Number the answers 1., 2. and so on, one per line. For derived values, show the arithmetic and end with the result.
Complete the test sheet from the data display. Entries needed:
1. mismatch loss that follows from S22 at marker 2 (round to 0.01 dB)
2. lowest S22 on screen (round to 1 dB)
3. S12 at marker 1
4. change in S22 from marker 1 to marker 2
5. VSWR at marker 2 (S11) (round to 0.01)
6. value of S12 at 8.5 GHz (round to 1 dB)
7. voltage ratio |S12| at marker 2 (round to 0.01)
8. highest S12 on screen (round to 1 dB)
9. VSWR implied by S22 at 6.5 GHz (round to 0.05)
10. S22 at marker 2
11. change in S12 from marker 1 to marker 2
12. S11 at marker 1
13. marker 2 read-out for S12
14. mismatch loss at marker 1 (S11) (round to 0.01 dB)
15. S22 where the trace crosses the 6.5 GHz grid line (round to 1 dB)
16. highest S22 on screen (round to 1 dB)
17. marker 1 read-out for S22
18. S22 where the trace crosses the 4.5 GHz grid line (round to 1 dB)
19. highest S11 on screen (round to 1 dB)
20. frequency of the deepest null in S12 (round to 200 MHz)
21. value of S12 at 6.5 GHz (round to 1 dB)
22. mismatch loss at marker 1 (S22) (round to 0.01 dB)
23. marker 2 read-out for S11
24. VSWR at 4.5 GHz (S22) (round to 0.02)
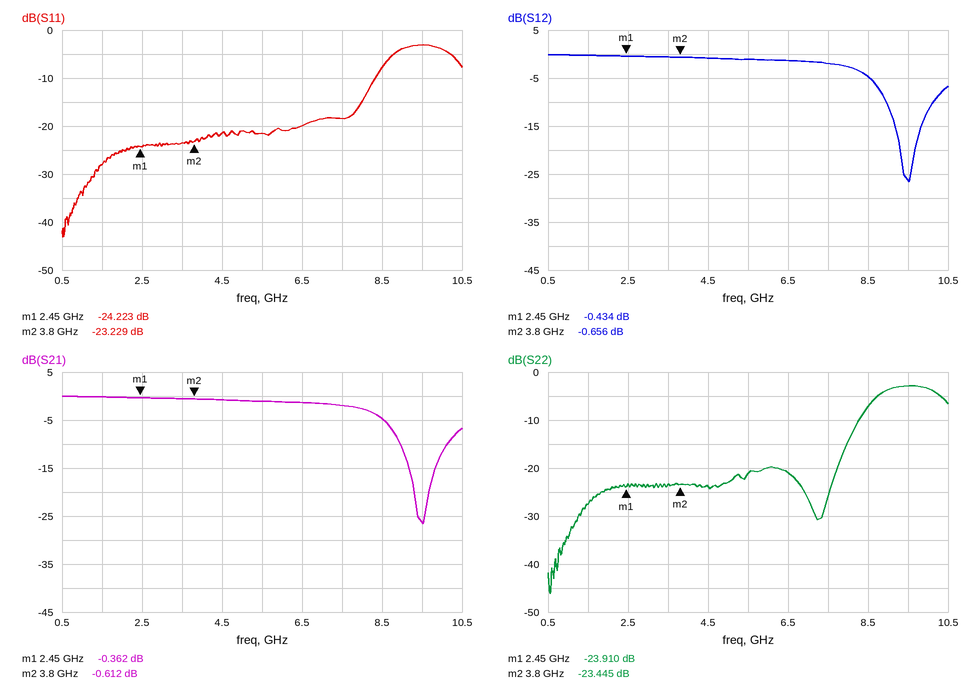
1. −10 log10(1 − 10^(-23.445/10)) ≈ 0.02 dB
2. -46 dB
3. -0.434 dB
4. -23.445 − (-23.91) = 0.465 dB
5. (1 + 0.0690)/(1 − 0.0690) ≈ 1.15
6. -5 dB
7. 10^(-0.656/20) ≈ 0.93
8. 0 dB
9. |Γ| = 10^(-21/20) = 0.0891; VSWR = (1 + 0.0891)/(1 − 0.0891) ≈ 1.20
10. -23.445 dB
11. -0.656 − (-0.434) = -0.222 dB
12. -24.223 dB
13. -0.656 dB
14. −10 log10(1 − 10^(-24.223/10)) ≈ 0.02 dB
15. -21 dB
16. -3 dB
17. -23.910 dB
18. -24 dB
19. -3 dB
20. 9.6 GHz
21. -1 dB
22. −10 log10(1 − 10^(-23.91/10)) ≈ 0.02 dB
23. -23.229 dB
24. |Γ| = 10^(-24/20) = 0.0631; VSWR = (1 + 0.0631)/(1 − 0.0631) ≈ 1.13, so 1.14 to the nearest 0.02
